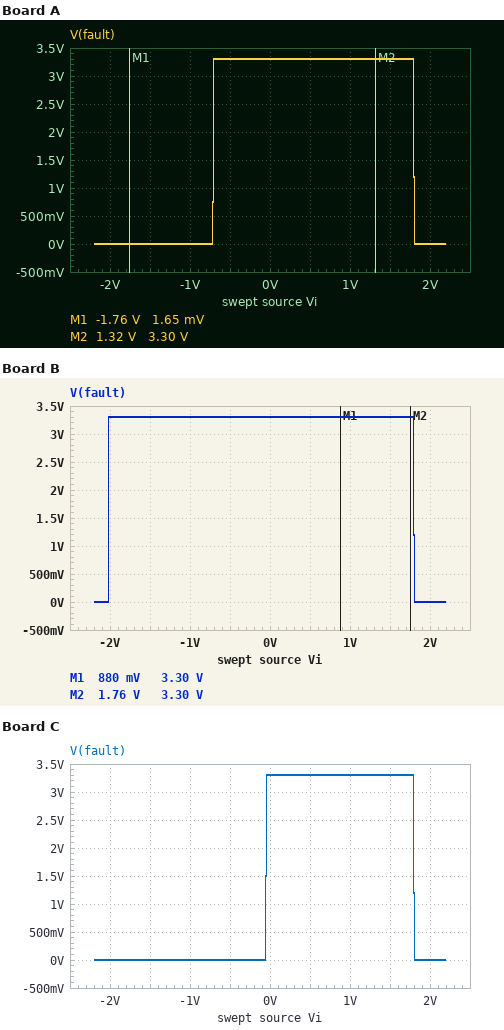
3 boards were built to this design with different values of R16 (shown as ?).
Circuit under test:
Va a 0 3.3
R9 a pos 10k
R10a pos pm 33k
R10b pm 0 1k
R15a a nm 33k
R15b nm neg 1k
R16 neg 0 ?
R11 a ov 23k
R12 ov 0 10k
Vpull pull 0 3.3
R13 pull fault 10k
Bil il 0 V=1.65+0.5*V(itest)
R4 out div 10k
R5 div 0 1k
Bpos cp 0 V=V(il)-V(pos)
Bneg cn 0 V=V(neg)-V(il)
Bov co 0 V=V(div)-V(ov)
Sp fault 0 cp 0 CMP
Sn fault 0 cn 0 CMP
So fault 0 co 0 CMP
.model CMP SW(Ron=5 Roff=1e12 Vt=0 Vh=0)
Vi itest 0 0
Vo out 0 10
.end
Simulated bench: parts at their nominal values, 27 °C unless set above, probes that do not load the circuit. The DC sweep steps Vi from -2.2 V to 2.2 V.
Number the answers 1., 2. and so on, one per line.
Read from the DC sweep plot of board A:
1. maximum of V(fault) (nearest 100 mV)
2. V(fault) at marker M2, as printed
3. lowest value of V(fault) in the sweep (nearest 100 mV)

1. 3.3 V
2. 3.30 V
3. 0 V
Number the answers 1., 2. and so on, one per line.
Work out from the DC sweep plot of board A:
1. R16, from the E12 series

1. 22 kΩ
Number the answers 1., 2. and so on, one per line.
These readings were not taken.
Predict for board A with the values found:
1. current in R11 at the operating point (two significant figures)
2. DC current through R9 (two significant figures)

1. 100 µA
2. 75 µA
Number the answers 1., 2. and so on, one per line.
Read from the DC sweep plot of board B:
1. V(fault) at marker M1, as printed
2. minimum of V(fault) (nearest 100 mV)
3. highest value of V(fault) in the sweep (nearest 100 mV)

1. 3.30 V
2. 0 V
3. 3.3 V
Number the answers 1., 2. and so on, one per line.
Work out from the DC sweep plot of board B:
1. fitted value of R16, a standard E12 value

1. 8.2 kΩ
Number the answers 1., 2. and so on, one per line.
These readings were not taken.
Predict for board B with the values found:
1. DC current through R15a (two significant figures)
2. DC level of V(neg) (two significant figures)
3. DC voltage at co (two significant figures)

1. 78 µA
2. 640 mV
3. -91 mV
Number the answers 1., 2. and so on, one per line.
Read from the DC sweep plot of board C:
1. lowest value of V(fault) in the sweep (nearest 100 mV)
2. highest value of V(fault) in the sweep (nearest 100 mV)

1. 0 V
2. 3.3 V
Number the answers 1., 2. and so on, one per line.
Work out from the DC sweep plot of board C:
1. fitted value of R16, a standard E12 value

1. 33 kΩ
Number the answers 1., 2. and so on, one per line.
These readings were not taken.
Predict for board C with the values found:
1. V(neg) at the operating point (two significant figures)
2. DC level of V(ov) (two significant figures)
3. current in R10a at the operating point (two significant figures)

1. 1.6 V
2. 1.0 V
3. 75 µA
